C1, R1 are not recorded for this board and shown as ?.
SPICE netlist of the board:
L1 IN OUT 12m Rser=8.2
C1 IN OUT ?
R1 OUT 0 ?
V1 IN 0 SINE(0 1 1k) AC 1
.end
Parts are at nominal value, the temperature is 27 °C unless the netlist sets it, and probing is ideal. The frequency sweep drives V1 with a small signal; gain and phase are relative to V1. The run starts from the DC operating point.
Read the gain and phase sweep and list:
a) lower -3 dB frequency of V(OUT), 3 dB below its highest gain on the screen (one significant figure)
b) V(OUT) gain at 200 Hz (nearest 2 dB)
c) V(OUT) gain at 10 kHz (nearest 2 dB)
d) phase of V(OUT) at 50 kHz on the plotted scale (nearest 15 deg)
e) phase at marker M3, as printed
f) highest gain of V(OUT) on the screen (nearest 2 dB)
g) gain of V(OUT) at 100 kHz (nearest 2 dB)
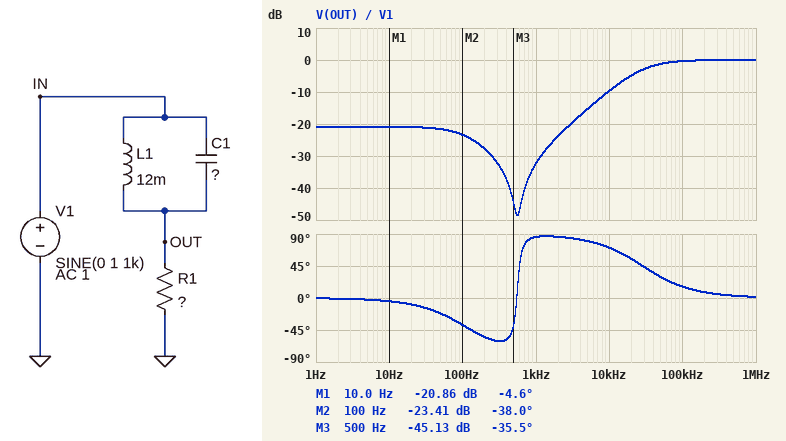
30 kHz
-28 dB
-10 dB
30 deg
-35.5 deg
0 dB
0 dB
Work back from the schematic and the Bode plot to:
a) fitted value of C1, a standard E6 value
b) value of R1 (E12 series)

6.8 µF
0.82 Ω
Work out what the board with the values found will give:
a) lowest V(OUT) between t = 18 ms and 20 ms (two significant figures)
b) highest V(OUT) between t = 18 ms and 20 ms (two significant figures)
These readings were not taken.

-24 mV
24 mV
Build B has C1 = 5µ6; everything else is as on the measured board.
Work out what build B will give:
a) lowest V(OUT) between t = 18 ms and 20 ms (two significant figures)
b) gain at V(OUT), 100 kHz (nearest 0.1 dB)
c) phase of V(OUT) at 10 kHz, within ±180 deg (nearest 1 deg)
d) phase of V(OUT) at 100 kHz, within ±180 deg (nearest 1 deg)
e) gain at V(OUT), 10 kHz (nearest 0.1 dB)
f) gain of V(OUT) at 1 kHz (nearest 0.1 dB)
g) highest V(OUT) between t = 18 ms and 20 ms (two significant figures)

-18 mV
-0.5 dB
74 deg
19 deg
-11.2 dB
-34.8 dB
18 mV
